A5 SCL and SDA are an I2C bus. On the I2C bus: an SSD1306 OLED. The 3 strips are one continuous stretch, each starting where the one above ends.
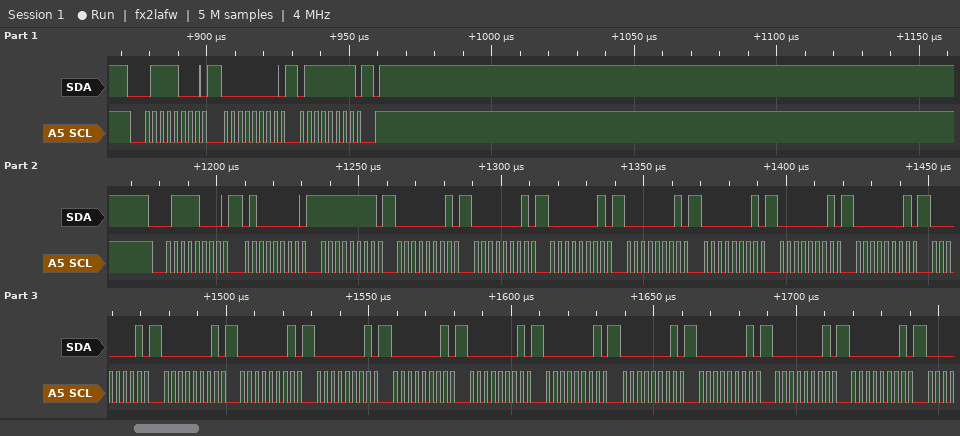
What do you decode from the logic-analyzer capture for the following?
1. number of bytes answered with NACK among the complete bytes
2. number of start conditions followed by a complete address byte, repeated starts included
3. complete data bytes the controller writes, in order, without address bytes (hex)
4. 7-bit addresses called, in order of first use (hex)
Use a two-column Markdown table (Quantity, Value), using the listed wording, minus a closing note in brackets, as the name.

| Quantity | Value |
|---|---|
| number of bytes answered with NACK among the complete bytes | 0 |
| number of start conditions followed by a complete address byte, repeated starts included | 2 |
| complete data bytes the controller writes, in order, without address bytes | 00 7F 40 FF 01 01 01 01 01 01 01 01 01 01 01 01 01 01 01 01 01 01 |
| 7-bit addresses called, in order of first use | 0x3C |
